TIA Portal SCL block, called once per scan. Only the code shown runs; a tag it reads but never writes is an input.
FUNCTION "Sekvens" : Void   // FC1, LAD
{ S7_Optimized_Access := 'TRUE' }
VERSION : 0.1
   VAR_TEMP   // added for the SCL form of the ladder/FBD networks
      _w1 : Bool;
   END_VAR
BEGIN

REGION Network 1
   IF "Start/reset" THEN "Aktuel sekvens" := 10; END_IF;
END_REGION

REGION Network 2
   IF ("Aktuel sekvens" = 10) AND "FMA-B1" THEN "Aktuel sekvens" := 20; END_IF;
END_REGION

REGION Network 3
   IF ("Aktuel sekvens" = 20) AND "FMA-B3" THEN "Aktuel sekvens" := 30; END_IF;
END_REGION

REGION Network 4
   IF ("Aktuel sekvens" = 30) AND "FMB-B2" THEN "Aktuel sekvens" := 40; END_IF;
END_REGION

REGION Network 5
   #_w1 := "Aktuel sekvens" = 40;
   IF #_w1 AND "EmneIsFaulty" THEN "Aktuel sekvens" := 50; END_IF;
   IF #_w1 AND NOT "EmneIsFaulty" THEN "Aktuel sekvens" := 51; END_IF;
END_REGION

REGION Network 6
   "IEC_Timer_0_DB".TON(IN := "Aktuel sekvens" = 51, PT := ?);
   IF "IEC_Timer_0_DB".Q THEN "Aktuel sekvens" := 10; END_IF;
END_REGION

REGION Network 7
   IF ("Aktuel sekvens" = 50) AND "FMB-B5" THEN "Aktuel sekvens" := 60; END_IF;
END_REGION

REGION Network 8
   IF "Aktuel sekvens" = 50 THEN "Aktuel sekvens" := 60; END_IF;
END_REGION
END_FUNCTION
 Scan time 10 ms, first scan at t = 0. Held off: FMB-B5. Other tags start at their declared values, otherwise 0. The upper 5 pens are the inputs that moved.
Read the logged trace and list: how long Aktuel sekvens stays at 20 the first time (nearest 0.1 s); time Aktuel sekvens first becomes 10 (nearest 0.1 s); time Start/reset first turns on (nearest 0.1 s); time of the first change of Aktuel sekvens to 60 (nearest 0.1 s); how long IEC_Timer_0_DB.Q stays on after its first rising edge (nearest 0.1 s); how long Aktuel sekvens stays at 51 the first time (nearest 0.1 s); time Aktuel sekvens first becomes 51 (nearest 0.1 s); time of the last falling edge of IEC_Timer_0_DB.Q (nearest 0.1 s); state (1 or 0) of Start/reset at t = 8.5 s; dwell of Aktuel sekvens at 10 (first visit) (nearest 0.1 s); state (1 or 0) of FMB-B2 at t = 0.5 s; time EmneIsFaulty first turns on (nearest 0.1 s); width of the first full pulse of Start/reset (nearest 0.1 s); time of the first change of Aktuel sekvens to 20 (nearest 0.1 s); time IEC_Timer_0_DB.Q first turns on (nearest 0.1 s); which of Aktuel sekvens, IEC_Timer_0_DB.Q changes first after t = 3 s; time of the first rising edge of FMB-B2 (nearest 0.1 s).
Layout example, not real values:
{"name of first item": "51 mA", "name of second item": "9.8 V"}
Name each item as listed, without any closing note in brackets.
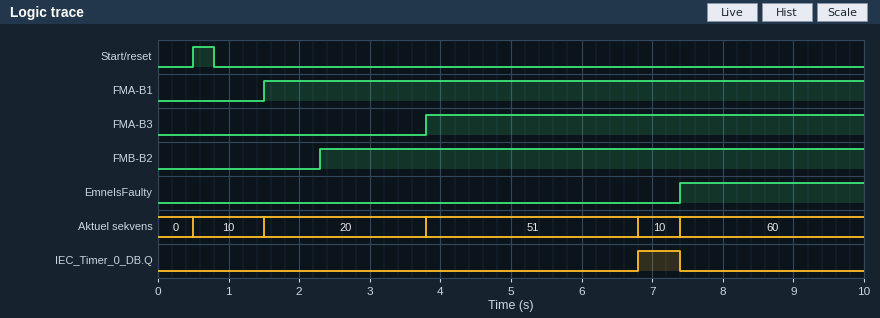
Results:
{"how long Aktuel sekvens stays at 20 the first time": "2.3 s", "time Aktuel sekvens first becomes 10": "0.5 s", "time Start/reset first turns on": "0.5 s", "time of the first change of Aktuel sekvens to 60": "7.4 s", "how long IEC_Timer_0_DB.Q stays on after its first rising edge": "0.6 s", "how long Aktuel sekvens stays at 51 the first time": "3.0 s", "time Aktuel sekvens first becomes 51": "3.8 s", "time of the last falling edge of IEC_Timer_0_DB.Q": "7.4 s", "state (1 or 0) of Start/reset at t = 8.5 s": "0", "dwell of Aktuel sekvens at 10 (first visit)": "1.0 s", "state (1 or 0) of FMB-B2 at t = 0.5 s": "0", "time EmneIsFaulty first turns on": "7.4 s", "width of the first full pulse of Start/reset": "0.3 s", "time of the first change of Aktuel sekvens to 20": "1.5 s", "time IEC_Timer_0_DB.Q first turns on": "6.8 s", "which of Aktuel sekvens, IEC_Timer_0_DB.Q changes first after t = 3 s": "Aktuel sekvens", "time of the first rising edge of FMB-B2": "2.3 s"}
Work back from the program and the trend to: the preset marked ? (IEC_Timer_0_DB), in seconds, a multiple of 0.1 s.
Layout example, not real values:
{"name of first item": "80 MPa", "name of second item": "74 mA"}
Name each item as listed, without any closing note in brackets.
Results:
{"the preset marked ? (IEC_Timer_0_DB), in seconds, a multiple of 0.1 s": "3.0 s"}
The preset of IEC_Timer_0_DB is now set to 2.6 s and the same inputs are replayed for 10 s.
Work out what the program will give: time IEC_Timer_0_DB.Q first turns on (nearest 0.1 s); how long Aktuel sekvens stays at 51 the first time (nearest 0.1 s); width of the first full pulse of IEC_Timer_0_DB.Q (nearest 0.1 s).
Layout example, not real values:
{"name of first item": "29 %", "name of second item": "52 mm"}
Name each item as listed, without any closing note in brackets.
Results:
{"time IEC_Timer_0_DB.Q first turns on": "6.4 s", "how long Aktuel sekvens stays at 51 the first time": "2.6 s", "width of the first full pulse of IEC_Timer_0_DB.Q": "1.0 s"}
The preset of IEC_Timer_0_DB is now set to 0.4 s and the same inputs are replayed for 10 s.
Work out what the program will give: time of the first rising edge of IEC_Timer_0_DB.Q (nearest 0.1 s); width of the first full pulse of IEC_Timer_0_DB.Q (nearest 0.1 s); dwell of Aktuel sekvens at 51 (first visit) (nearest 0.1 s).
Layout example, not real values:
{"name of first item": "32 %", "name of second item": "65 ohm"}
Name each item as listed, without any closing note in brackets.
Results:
{"time of the first rising edge of IEC_Timer_0_DB.Q": "4.2 s", "width of the first full pulse of IEC_Timer_0_DB.Q": "3.2 s", "dwell of Aktuel sekvens at 51 (first visit)": "0.4 s"}
